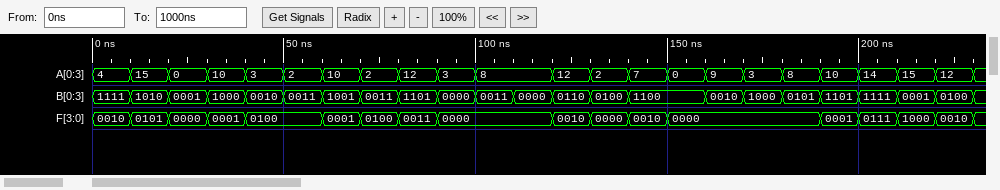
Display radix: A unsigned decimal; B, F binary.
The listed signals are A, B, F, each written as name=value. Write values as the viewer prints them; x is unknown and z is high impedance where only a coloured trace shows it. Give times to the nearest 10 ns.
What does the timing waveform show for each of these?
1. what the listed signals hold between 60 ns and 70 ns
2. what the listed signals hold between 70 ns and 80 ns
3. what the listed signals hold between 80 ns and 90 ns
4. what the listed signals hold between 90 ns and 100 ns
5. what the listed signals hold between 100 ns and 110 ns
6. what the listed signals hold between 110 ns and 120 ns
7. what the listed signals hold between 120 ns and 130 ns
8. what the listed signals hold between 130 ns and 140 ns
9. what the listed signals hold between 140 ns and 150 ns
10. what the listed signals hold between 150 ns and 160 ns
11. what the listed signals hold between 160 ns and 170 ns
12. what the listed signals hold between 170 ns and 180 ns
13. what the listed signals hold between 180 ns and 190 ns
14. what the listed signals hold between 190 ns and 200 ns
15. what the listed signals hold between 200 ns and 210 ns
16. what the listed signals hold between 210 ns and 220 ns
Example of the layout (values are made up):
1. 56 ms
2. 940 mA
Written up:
1. A=10, B=1001, F=0001
2. A=2, B=0011, F=0100
3. A=12, B=1101, F=0011
4. A=3, B=0000, F=0000
5. A=8, B=0011, F=0000
6. A=8, B=0000, F=0000
7. A=12, B=0110, F=0010
8. A=2, B=0100, F=0000
9. A=7, B=1100, F=0010
10. A=0, B=1100, F=0000
11. A=9, B=0010, F=0000
12. A=3, B=1000, F=0000
13. A=8, B=0101, F=0000
14. A=10, B=1101, F=0001
15. A=14, B=1111, F=0111
16. A=15, B=0001, F=1000
